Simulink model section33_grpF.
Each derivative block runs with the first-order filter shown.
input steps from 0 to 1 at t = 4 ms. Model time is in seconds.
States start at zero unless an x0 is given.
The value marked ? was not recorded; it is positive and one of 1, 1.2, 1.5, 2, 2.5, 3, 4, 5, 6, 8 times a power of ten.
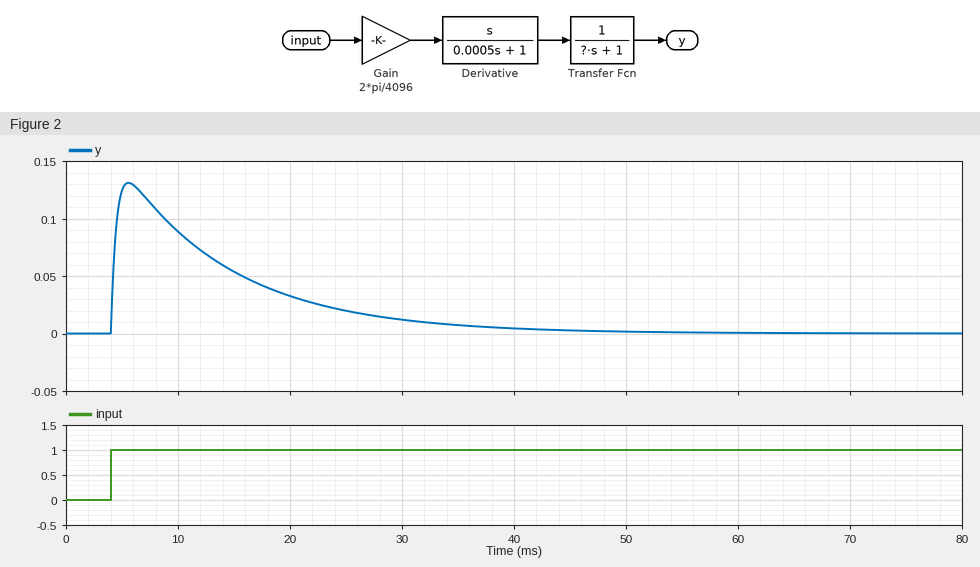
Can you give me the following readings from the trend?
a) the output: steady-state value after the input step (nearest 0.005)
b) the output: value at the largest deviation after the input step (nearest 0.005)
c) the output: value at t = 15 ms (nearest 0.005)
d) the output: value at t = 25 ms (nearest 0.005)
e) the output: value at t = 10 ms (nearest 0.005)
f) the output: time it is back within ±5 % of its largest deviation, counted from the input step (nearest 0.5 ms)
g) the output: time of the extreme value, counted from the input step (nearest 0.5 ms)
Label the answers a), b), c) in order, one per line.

a) 0.000
b) 0.130
c) 0.055
d) 0.020
e) 0.090
f) 32.0 ms
g) 1.5 ms
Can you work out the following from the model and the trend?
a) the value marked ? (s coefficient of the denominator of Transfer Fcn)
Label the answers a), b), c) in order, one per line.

a) 0.01
